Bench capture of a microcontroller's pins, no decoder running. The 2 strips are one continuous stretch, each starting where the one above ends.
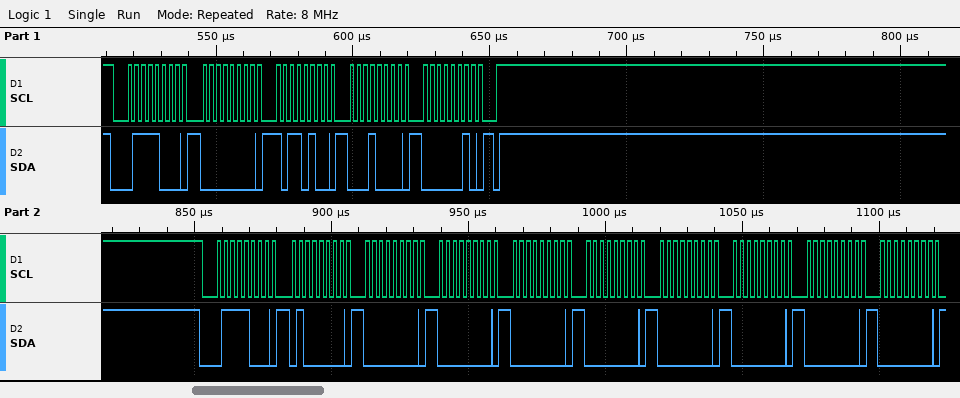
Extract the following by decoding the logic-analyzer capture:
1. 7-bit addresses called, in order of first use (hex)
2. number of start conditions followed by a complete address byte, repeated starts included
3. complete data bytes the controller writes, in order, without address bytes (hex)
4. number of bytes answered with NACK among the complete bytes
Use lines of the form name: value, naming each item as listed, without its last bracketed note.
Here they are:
7-bit addresses called, in order of first use: 0x3C
number of start conditions followed by a complete address byte, repeated starts included: 2
complete data bytes the controller writes, in order, without address bytes: 00 B4 10 02 40 00 00 00 00 00 00 00 00
number of bytes answered with NACK among the complete bytes: 0
